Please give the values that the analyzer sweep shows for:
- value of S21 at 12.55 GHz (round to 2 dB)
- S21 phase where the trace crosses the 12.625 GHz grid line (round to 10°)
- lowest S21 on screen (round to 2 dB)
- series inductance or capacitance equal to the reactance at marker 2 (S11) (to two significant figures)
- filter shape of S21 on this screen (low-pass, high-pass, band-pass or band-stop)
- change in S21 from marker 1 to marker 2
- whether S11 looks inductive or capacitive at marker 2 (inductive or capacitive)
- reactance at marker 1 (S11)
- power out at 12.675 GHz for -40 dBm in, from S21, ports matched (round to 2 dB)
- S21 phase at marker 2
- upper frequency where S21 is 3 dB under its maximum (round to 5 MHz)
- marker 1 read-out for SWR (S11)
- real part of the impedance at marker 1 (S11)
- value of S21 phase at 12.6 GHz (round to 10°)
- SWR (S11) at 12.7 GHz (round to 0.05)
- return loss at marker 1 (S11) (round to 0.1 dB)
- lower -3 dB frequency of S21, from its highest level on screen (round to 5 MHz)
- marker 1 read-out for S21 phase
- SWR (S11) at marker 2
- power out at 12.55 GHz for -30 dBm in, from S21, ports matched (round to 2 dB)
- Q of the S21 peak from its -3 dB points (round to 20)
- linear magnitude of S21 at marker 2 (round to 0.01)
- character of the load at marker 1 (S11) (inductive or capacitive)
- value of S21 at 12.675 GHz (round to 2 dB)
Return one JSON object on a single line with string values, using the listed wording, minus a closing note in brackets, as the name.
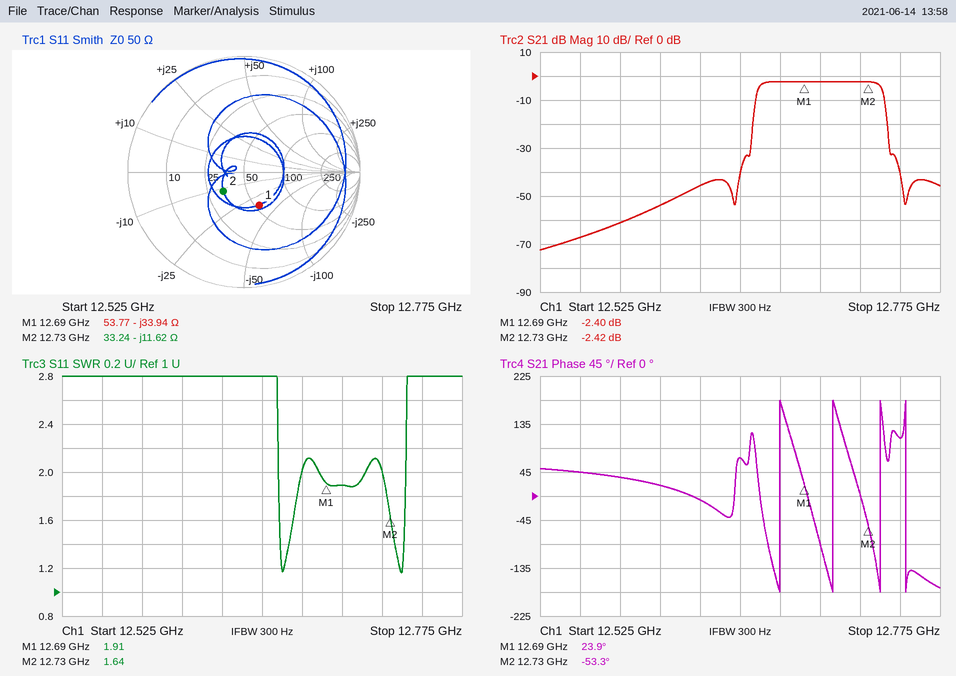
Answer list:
{"value of S21 at 12.55 GHz": "-68 dB", "S21 phase where the trace crosses the 12.625 GHz grid line": "-10°", "lowest S21 on screen": "-72 dB", "series inductance or capacitance equal to the reactance at marker 2 (S11)": "1.1 pF", "filter shape of S21 on this screen": "band-pass", "change in S21 from marker 1 to marker 2": "-0.02 dB", "whether S11 looks inductive or capacitive at marker 2": "capacitive", "reactance at marker 1": "-33.94 Ω", "power out at 12.675 GHz for -40 dBm in, from S21, ports matched": "-42 dBm", "S21 phase at marker 2": "-53.3°", "upper frequency where S21 is 3 dB under its maximum": "12.740 GHz", "marker 1 read-out for SWR": "1.91", "real part of the impedance at marker 1": "53.77 Ω", "value of S21 phase at 12.6 GHz": "20°", "SWR (S11) at 12.7 GHz": "1.90", "return loss at marker 1 (S11)": "10.1 dB", "lower -3 dB frequency of S21, from its highest level on screen": "12.660 GHz", "marker 1 read-out for S21 phase": "23.9°", "SWR (S11) at marker 2": "1.64", "power out at 12.55 GHz for -30 dBm in, from S21, ports matched": "-98 dBm", "Q of the S21 peak from its -3 dB points": "160", "linear magnitude of S21 at marker 2": "0.76", "character of the load at marker 1 (S11)": "capacitive", "value of S21 at 12.675 GHz": "-2 dB"}
